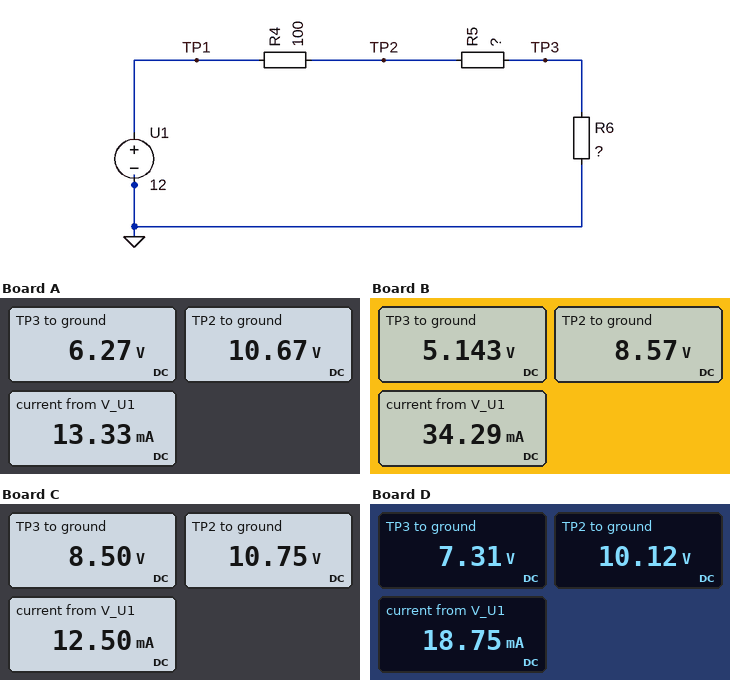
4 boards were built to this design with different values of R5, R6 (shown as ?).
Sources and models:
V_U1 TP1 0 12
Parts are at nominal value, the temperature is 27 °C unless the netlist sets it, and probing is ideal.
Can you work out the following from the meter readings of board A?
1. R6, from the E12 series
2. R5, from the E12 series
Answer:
470 Ω
330 Ω
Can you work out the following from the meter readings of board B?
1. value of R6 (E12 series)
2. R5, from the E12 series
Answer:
150 Ω
100 Ω
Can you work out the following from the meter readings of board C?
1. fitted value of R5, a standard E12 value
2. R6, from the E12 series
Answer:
180 Ω
680 Ω
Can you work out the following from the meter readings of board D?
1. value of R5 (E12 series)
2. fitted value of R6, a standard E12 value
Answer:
150 Ω
390 Ω
